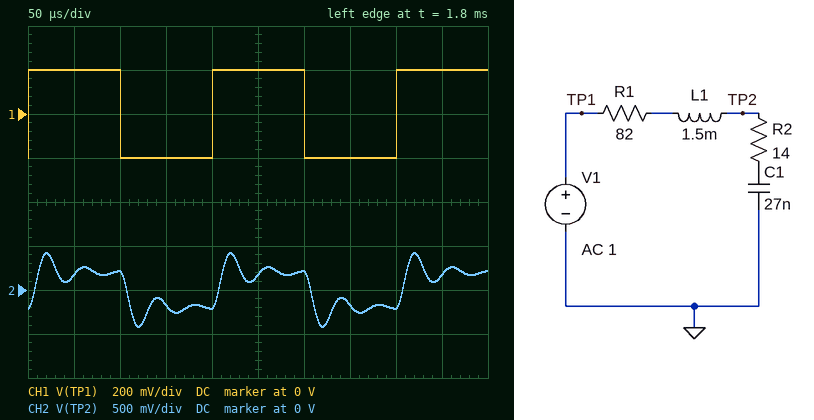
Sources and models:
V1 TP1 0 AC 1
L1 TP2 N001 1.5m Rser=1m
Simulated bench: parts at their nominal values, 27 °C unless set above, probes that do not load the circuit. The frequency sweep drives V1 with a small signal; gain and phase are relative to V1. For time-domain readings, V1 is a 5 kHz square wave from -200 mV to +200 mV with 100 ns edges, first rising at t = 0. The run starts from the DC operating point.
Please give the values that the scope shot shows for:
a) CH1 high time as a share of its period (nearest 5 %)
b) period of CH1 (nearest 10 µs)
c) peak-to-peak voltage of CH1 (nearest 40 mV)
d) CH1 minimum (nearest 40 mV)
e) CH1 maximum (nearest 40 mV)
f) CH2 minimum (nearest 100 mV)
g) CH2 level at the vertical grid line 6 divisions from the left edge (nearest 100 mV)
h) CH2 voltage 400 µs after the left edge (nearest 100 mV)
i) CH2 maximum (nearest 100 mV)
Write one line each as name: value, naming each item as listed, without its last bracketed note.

CH1 high time as a share of its period: 50 %
period of CH1: 200 µs
peak-to-peak voltage of CH1: 400 mV
CH1 minimum: -200 mV
CH1 maximum: 200 mV
CH2 minimum: -400 mV
CH2 level at the vertical grid line 6 divisions from the left edge: 200 mV
CH2 voltage 400 µs after the left edge: -200 mV
CH2 maximum: 400 mV
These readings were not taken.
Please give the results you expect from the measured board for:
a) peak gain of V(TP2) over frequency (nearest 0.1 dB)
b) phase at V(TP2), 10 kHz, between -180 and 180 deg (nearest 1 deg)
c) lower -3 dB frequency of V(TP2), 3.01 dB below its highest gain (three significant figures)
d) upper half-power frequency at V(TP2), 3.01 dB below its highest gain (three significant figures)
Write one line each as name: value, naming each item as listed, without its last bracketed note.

peak gain of V(TP2) over frequency: 8.0 dB
phase at V(TP2), 10 kHz, between -180 and 180 deg: -10 deg
lower -3 dB frequency of V(TP2), 3.01 dB below its highest gain: 18.0 kHz
upper half-power frequency at V(TP2), 3.01 dB below its highest gain: 28.7 kHz
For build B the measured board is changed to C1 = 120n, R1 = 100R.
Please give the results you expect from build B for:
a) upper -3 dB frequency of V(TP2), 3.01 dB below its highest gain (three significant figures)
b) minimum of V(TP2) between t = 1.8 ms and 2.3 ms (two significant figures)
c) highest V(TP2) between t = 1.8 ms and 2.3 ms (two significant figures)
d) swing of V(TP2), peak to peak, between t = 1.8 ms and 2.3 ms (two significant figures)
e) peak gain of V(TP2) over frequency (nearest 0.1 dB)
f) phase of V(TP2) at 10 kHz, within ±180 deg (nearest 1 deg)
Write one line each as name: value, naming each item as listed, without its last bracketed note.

upper -3 dB frequency of V(TP2), 3.01 dB below its highest gain: 13.9 kHz
minimum of V(TP2) between t = 1.8 ms and 2.3 ms: -260 mV
highest V(TP2) between t = 1.8 ms and 2.3 ms: 260 mV
swing of V(TP2), peak to peak, between t = 1.8 ms and 2.3 ms: 520 mV
peak gain of V(TP2) over frequency: 1.2 dB
phase of V(TP2) at 10 kHz, within ±180 deg: -65 deg
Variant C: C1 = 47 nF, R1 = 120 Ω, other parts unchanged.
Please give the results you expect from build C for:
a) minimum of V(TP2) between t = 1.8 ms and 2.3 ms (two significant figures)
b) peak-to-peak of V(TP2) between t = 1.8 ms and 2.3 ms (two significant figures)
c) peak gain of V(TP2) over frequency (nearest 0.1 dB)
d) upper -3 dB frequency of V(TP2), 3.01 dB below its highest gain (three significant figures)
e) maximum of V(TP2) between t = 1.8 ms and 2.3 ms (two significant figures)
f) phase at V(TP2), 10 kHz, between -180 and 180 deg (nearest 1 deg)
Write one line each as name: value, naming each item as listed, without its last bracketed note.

minimum of V(TP2) between t = 1.8 ms and 2.3 ms: -310 mV
peak-to-peak of V(TP2) between t = 1.8 ms and 2.3 ms: 630 mV
peak gain of V(TP2) over frequency: 3.2 dB
upper -3 dB frequency of V(TP2), 3.01 dB below its highest gain: 22.6 kHz
maximum of V(TP2) between t = 1.8 ms and 2.3 ms: 310 mV
phase at V(TP2), 10 kHz, between -180 and 180 deg: -26 deg
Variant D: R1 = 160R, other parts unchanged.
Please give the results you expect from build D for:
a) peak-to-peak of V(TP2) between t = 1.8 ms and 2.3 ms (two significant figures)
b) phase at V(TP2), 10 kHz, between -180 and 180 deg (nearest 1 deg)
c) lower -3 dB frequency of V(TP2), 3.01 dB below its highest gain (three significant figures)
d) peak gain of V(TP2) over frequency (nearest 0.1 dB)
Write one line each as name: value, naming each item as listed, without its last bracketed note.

peak-to-peak of V(TP2) between t = 1.8 ms and 2.3 ms: 630 mV
phase at V(TP2), 10 kHz, between -180 and 180 deg: -18 deg
lower -3 dB frequency of V(TP2), 3.01 dB below its highest gain: 5.19 kHz
peak gain of V(TP2) over frequency: 3.3 dB
